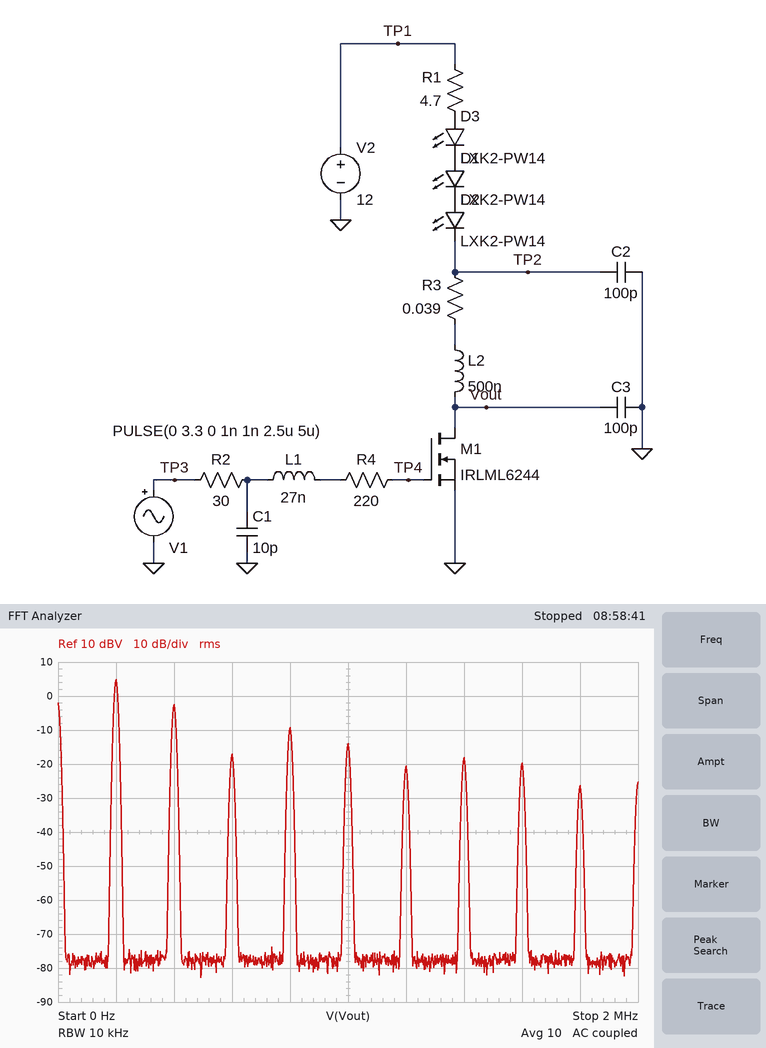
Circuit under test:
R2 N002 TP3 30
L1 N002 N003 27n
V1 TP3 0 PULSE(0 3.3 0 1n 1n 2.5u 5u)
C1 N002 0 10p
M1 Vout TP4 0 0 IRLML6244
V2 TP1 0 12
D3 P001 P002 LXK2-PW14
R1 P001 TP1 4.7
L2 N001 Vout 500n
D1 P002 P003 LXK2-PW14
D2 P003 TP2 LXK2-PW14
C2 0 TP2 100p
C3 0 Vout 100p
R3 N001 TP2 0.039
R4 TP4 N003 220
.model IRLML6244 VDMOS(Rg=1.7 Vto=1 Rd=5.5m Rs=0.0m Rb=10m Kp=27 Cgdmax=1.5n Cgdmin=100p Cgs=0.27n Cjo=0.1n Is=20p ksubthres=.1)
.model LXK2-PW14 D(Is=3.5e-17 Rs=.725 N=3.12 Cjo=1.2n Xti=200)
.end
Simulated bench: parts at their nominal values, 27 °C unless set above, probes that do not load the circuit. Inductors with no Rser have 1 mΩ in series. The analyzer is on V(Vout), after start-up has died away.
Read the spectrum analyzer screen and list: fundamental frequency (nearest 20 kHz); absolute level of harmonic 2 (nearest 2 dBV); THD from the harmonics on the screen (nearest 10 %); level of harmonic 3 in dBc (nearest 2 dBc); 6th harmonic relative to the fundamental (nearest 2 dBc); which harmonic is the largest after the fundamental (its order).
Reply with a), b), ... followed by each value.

a) 200 kHz
b) -2 dBV
c) 50 %
d) -22 dBc
e) -26 dBc
f) 2
